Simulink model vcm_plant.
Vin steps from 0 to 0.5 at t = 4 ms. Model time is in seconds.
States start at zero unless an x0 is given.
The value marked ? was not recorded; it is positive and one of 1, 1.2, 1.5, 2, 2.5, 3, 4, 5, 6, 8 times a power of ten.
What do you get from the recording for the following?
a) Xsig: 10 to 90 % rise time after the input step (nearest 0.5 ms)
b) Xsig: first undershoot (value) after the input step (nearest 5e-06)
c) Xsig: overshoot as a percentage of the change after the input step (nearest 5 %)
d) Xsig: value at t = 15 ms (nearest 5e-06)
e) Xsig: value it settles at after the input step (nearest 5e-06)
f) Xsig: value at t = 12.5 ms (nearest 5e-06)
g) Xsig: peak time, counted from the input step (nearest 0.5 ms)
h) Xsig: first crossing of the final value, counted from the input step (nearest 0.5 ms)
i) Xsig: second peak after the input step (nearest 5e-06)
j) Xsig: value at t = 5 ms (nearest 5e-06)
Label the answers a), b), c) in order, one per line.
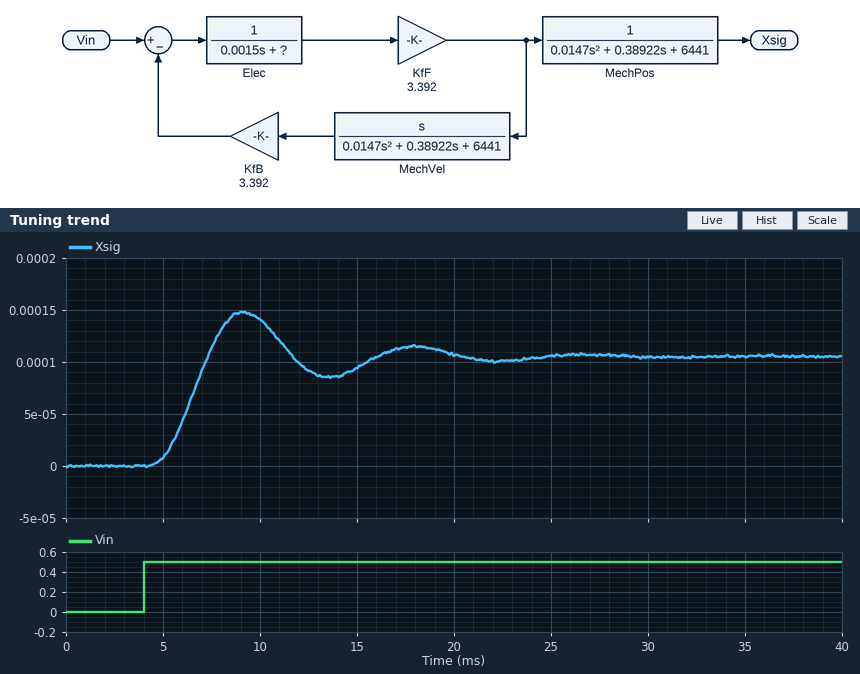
a) 2.0 ms
b) 0.000085
c) 40 %
d) 0.000095
e) 0.000105
f) 0.000090
g) 5.0 ms
h) 3.5 ms
i) 0.000115
j) 0.000010
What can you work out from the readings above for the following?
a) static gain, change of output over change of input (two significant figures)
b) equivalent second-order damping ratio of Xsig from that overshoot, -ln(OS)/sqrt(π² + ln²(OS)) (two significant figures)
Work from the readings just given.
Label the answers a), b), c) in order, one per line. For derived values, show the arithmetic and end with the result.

a) (0.000105 - 0) / (0.5 - 0) = 0.00021
b) ln(0.4) = -0.916; 0.916 / sqrt(9.870 + 0.840) = 0.28
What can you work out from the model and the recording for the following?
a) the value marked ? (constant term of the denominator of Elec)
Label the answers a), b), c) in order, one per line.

a) 2.5
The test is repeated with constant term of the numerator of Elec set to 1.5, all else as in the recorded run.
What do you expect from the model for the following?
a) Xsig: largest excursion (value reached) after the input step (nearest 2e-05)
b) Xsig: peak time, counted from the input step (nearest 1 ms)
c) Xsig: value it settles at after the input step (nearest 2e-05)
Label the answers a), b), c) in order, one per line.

a) 0.00020
b) 5 ms
c) 0.00016
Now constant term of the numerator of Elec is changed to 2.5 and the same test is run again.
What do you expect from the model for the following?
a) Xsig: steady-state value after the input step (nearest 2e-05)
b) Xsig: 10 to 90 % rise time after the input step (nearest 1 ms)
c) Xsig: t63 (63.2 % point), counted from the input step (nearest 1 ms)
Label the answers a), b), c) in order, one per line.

a) 0.00026
b) 3 ms
c) 3 ms
